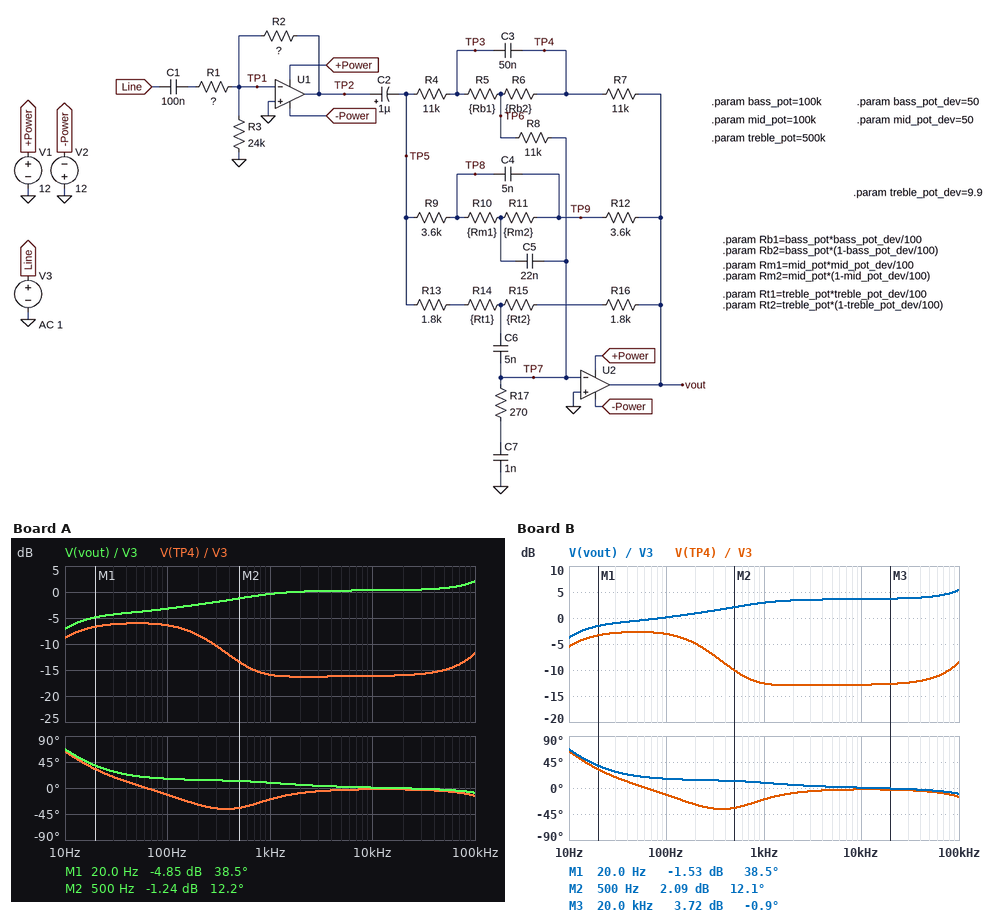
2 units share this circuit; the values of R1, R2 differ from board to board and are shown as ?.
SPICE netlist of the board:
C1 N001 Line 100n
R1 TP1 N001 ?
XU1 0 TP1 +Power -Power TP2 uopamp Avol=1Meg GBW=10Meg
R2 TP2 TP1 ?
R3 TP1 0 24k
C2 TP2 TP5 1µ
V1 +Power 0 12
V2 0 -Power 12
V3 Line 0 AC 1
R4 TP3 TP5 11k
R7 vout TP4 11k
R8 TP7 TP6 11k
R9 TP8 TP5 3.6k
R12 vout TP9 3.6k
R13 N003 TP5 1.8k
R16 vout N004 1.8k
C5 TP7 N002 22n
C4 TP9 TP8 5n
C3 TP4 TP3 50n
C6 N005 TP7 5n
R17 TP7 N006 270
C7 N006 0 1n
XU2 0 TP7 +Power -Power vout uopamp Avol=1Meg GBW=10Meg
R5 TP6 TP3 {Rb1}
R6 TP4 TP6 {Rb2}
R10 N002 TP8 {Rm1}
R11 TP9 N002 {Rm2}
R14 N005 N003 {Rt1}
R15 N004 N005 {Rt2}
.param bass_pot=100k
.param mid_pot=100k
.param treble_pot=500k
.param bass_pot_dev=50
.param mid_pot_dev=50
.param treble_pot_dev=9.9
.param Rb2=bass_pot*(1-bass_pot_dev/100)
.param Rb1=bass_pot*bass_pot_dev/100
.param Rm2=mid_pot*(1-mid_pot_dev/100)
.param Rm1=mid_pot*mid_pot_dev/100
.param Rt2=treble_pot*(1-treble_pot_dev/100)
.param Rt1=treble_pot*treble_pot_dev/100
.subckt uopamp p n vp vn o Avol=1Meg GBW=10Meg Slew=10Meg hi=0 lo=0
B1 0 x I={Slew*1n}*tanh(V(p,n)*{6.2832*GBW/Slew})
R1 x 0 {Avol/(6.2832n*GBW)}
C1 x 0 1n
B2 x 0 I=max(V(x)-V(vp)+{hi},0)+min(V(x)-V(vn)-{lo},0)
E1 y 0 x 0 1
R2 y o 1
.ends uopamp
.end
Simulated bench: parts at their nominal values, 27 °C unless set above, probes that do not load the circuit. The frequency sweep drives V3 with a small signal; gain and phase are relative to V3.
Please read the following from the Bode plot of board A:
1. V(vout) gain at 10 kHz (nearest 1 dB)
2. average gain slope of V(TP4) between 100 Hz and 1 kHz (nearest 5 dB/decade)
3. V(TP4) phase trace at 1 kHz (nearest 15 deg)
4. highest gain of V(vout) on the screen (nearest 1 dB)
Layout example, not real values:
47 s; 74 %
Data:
0 dB; -10 dB/decade; -15 deg; 2 dB
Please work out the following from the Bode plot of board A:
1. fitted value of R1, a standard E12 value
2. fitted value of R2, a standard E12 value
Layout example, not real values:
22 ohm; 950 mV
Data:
220 kΩ; 150 kΩ
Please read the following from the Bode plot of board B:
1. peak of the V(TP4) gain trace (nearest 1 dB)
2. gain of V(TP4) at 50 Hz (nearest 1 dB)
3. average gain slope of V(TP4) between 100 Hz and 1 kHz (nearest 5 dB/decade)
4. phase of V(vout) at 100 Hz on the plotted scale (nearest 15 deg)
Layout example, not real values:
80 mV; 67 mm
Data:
-3 dB; -3 dB; -10 dB/decade; 15 deg
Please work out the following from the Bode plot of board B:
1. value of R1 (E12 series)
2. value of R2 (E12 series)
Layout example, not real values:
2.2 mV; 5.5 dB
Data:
220 kΩ; 220 kΩ
